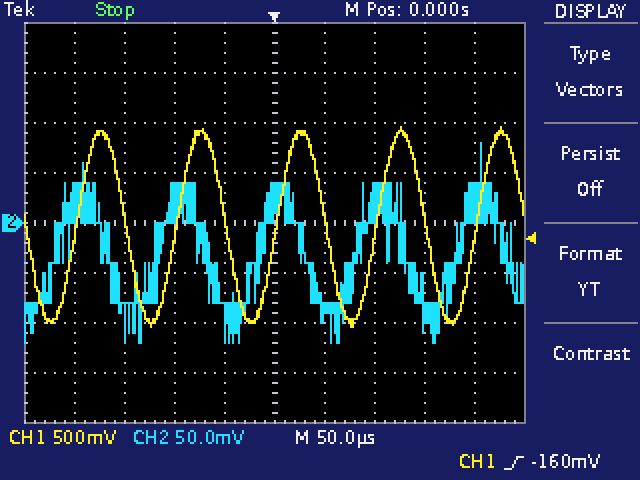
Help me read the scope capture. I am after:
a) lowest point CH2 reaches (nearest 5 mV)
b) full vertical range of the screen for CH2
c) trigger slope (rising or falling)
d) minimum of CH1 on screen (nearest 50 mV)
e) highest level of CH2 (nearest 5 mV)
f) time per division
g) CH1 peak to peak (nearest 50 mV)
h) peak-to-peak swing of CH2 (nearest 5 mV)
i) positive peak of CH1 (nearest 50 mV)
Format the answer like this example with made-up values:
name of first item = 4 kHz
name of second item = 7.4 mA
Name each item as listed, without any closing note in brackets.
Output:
lowest point CH2 reaches = -120 mV
full vertical range of the screen for CH2 = 400 mV
trigger slope = rising
minimum of CH1 on screen = -1.05 V
highest level of CH2 = 80 mV
time per division = 50 µs
CH1 peak to peak = 2.00 V
peak-to-peak swing of CH2 = 200 mV
positive peak of CH1 = 950 mV
